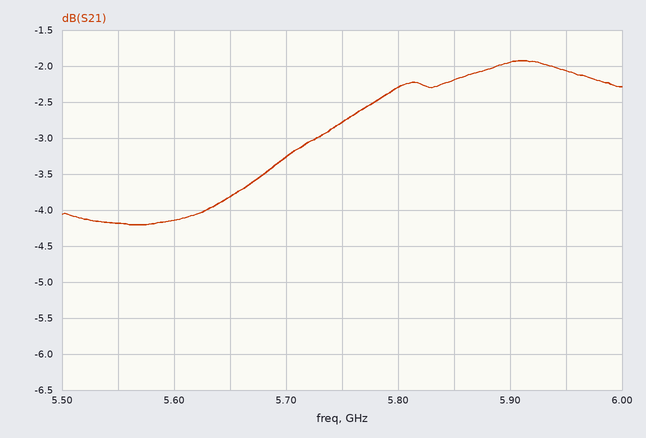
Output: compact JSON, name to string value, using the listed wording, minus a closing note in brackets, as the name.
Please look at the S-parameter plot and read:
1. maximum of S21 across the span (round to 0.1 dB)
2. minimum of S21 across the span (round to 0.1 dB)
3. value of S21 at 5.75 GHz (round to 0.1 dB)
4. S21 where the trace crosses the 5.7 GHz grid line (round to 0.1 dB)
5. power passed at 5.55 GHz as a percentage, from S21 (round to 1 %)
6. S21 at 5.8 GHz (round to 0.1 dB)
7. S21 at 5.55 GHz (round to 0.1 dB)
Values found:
{"maximum of S21 across the span": "-1.9 dB", "minimum of S21 across the span": "-4.2 dB", "value of S21 at 5.75 GHz": "-2.8 dB", "S21 where the trace crosses the 5.7 GHz grid line": "-3.3 dB", "power passed at 5.55 GHz as a percentage, from S21": "38 %", "S21 at 5.8 GHz": "-2.3 dB", "S21 at 5.55 GHz": "-4.2 dB"}
